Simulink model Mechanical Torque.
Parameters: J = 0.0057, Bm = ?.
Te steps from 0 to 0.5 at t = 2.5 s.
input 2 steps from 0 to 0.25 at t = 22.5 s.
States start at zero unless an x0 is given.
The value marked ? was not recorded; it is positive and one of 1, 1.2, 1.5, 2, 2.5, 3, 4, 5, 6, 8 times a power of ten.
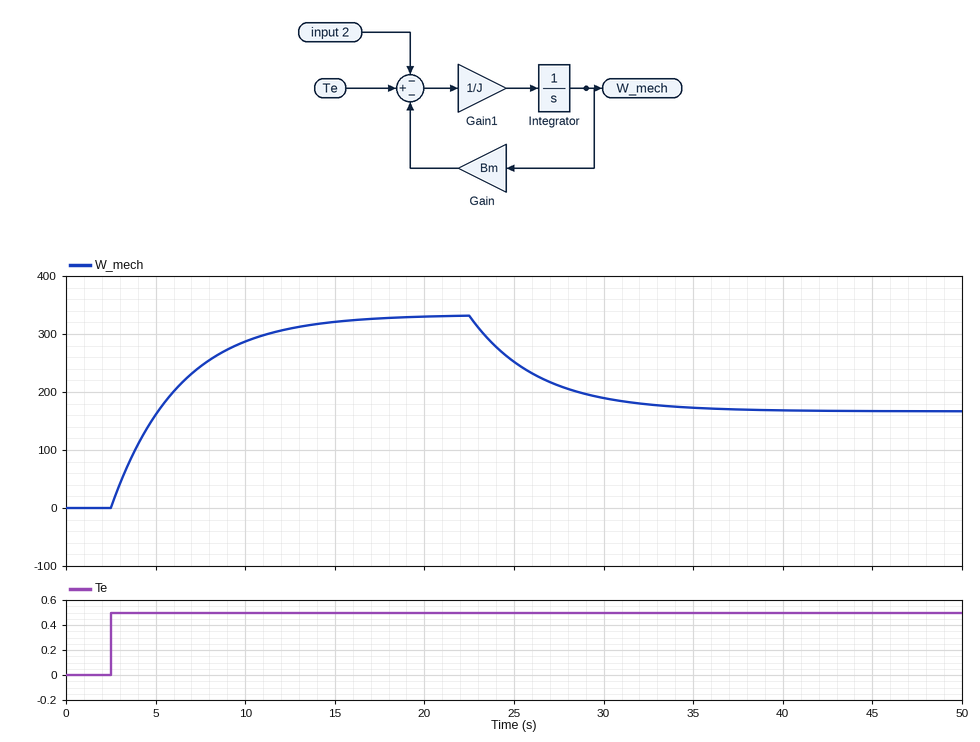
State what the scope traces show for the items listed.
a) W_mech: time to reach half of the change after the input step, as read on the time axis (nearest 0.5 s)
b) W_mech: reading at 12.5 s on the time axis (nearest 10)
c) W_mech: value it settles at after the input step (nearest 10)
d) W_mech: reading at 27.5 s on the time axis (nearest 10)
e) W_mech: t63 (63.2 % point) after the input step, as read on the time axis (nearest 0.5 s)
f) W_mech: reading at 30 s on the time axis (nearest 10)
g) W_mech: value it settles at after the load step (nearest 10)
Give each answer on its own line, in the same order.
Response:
5.0 s
310
330
210
6.5 s
190
170
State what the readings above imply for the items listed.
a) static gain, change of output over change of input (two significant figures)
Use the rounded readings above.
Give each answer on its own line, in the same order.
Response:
660
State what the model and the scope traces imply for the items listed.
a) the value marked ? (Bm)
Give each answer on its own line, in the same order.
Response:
0.0015
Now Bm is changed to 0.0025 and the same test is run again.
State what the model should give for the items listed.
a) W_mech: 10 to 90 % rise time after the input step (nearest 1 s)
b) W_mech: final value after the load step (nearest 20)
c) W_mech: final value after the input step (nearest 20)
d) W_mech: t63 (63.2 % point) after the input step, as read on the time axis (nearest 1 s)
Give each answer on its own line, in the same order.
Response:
5 s
100
200
5 s
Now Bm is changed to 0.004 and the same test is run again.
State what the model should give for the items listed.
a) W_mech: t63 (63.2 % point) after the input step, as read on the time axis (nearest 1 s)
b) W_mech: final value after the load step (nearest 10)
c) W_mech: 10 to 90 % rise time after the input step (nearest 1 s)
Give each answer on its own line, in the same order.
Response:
4 s
60
3 s
